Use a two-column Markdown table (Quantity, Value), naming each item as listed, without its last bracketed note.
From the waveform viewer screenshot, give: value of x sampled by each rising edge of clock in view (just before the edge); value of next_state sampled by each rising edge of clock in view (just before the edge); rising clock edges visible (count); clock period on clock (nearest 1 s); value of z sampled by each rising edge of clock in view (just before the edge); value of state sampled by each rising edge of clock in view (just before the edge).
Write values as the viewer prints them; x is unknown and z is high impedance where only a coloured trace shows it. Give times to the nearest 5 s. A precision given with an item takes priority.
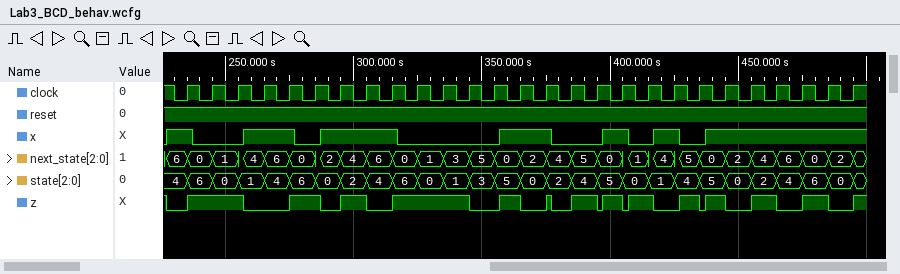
| Quantity | Value |
|---|---|
| value of x sampled by each rising edge of clock in view | 1 0 0 1 1 0 1 1 1 0 0 0 0 1 1 0 0 1 0 1 0 1 1 1 1 1 1 |
| value of next_state sampled by each rising edge of clock in view | 6, 0, 1, 4, 6, 0, 2, 4, 6, 0, 1, 3, 5, 0, 2, 4, 5, 0, 1, 4, 5, 0, 2, 4, 6, 0, 2 |
| rising clock edges visible | 27 |
| clock period on clock | 10 s |
| value of z sampled by each rising edge of clock in view | 0 1 1 0 0 1 0 1 0 1 1 1 0 1 0 0 1 1 1 0 1 1 0 1 0 1 0 |
| value of state sampled by each rising edge of clock in view | 4, 6, 0, 1, 4, 6, 0, 2, 4, 6, 0, 1, 3, 5, 0, 2, 4, 5, 0, 1, 4, 5, 0, 2, 4, 6, 0 |
